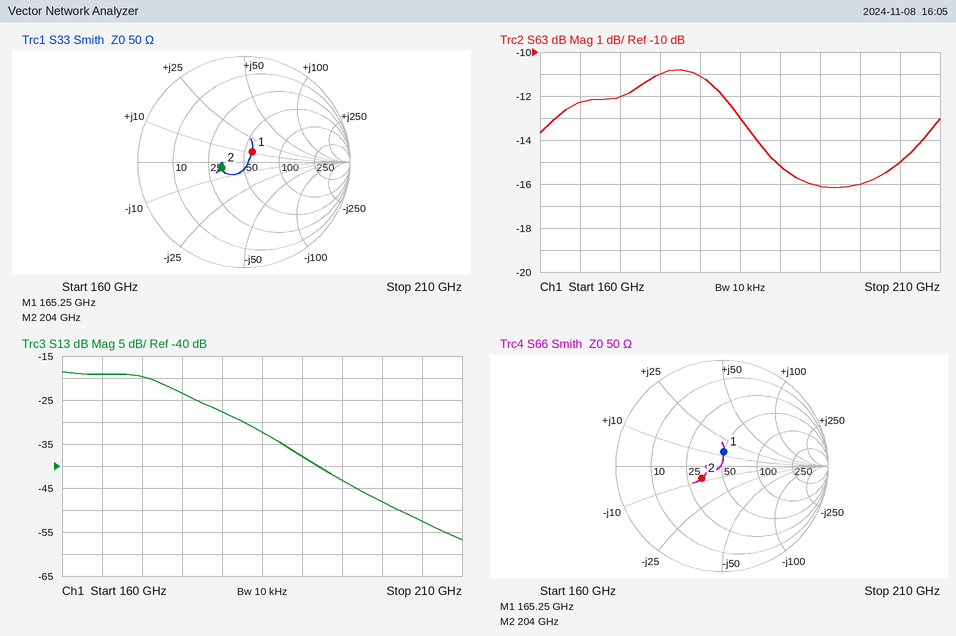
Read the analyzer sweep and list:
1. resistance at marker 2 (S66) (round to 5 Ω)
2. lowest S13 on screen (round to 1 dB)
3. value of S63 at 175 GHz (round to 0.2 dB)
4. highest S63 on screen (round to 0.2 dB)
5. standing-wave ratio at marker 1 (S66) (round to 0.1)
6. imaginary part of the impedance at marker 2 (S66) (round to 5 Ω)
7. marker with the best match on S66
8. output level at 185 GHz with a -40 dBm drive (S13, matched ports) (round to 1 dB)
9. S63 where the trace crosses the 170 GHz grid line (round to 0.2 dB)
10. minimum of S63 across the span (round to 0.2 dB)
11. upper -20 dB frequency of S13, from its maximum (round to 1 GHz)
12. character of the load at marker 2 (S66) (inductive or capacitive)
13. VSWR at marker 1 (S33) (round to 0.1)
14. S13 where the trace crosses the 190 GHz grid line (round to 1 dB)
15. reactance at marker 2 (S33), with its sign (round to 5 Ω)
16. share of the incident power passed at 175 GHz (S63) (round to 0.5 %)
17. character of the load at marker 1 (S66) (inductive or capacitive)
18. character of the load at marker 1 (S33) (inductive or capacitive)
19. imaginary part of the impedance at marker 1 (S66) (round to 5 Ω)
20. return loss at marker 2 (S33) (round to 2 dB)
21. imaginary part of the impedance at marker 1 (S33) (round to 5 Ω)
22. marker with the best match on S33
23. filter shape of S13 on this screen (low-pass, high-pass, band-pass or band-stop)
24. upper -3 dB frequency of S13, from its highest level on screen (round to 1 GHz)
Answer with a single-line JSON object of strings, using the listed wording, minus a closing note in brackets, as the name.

{"resistance at marker 2 (S66)": "35 Ω", "lowest S13 on screen": "-57 dB", "value of S63 at 175 GHz": "-11.0 dB", "highest S63 on screen": "-10.8 dB", "standing-wave ratio at marker 1 (S66)": "1.3", "imaginary part of the impedance at marker 2 (S66)": "-10 Ω", "marker with the best match on S66": "marker 1", "output level at 185 GHz with a -40 dBm drive (S13, matched ports)": "-72 dBm", "S63 where the trace crosses the 170 GHz grid line": "-12.0 dB", "minimum of S63 across the span": "-16.2 dB", "upper -20 dB frequency of S13, from its maximum": "191 GHz", "character of the load at marker 2 (S66)": "capacitive", "VSWR at marker 1 (S33)": "1.3", "S13 where the trace crosses the 190 GHz grid line": "-38 dB", "reactance at marker 2 (S33), with its sign": "-5 Ω", "share of the incident power passed at 175 GHz (S63)": "8.0 %", "character of the load at marker 1 (S66)": "inductive", "character of the load at marker 1 (S33)": "inductive", "imaginary part of the impedance at marker 1 (S66)": "+15 Ω", "return loss at marker 2 (S33)": "14 dB", "imaginary part of the impedance at marker 1 (S33)": "+10 Ω", "marker with the best match on S33": "marker 1", "filter shape of S13 on this screen": "low-pass", "upper -3 dB frequency of S13, from its highest level on screen": "173 GHz"}
